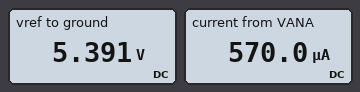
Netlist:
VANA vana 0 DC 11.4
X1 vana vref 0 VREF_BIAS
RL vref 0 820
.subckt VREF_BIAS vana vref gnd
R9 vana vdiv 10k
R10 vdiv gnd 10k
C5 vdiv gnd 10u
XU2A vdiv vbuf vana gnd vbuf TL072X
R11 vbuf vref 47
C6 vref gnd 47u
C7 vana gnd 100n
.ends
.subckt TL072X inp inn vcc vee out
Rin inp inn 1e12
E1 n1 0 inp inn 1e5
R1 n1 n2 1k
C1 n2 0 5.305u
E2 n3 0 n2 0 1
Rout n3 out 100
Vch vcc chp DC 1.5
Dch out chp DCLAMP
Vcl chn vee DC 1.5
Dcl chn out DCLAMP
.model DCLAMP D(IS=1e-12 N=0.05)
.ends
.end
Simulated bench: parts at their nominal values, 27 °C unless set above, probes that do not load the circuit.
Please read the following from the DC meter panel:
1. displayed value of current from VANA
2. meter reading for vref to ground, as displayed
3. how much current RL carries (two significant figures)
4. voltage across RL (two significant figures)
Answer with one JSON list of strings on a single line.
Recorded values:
["570.0 µA", "5.391 V", "6.6 mA", "5.4 V"]
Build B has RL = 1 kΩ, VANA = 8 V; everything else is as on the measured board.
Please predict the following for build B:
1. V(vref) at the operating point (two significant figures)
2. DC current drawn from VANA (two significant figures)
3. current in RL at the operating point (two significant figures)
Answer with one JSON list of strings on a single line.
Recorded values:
["3.8 V", "400 µA", "3.8 mA"]
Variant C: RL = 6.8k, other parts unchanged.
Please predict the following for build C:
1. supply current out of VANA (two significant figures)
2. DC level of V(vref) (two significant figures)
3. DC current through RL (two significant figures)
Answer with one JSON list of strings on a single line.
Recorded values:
["570 µA", "5.7 V", "830 µA"]
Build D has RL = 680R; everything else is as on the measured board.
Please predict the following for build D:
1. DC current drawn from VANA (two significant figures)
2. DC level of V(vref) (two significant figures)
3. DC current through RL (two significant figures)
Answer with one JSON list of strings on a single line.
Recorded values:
["570 µA", "5.3 V", "7.8 mA"]
